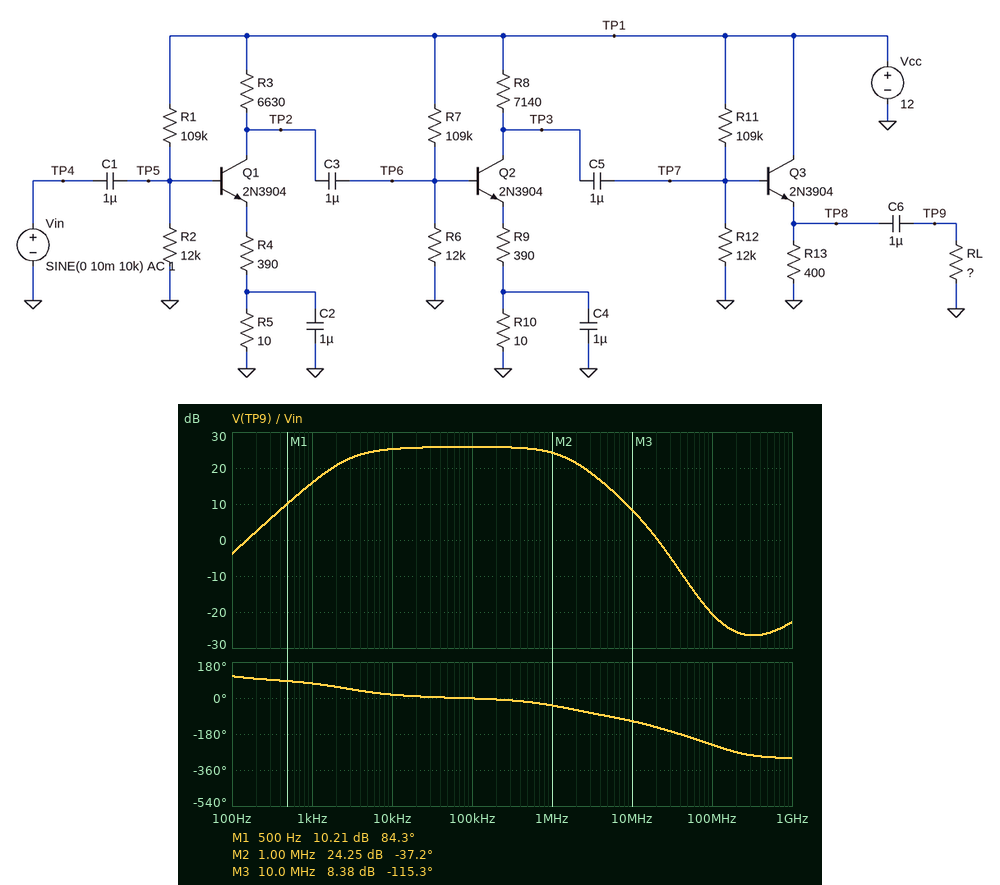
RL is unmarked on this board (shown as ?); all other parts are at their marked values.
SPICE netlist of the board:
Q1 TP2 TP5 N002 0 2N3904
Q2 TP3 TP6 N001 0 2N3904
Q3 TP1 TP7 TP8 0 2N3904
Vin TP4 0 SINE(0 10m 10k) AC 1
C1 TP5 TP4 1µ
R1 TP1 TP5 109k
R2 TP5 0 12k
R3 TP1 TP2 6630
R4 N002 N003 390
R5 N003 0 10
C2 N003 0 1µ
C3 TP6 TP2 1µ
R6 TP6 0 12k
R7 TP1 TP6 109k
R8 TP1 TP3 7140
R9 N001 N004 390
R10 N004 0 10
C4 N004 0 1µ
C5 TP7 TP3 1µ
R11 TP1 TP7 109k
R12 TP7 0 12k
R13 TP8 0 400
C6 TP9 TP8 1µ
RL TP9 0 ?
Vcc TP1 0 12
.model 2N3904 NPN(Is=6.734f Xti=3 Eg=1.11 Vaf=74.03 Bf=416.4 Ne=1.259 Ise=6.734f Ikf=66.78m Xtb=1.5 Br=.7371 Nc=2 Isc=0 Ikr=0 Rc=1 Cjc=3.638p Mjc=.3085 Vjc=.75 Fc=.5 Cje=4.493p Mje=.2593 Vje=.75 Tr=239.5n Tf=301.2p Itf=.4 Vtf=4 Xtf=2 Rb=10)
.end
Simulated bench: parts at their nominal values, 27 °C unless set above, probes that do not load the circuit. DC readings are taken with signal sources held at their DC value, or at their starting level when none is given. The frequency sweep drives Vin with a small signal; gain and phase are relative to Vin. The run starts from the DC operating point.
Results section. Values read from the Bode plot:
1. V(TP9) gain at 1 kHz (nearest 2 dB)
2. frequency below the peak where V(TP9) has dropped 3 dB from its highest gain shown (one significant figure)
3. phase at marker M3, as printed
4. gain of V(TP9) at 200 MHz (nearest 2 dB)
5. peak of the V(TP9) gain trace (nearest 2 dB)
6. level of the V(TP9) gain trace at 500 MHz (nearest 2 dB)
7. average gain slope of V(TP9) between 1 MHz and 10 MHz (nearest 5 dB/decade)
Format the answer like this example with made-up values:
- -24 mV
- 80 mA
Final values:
- 16 dB
- 3 kHz
- -115.3 deg
- -26 dB
- 26 dB
- -26 dB
- -15 dB/decade
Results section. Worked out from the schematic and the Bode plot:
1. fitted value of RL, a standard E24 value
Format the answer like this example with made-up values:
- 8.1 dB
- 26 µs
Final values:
- 13 Ω
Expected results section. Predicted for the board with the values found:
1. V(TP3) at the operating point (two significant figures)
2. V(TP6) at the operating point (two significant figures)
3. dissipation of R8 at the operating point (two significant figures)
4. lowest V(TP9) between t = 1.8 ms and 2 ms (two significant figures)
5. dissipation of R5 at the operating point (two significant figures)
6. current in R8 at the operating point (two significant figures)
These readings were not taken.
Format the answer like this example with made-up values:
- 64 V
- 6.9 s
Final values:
- 4.2 V
- 1.1 V
- 8.5 mW
- -32 mV
- 12 µW
- 1.1 mA
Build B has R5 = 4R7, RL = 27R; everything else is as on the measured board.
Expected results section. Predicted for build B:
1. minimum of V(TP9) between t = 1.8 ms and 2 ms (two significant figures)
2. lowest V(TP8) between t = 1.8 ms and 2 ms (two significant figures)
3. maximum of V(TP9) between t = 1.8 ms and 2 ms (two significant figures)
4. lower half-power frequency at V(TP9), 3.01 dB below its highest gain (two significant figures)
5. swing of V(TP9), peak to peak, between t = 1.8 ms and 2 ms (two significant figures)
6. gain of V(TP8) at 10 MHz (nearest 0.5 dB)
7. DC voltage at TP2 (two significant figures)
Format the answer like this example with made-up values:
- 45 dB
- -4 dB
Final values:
- -61 mV
- 790 mV
- 190 mV
- 2.4 kHz
- 250 mV
- 13.0 dB
- 4.7 V
